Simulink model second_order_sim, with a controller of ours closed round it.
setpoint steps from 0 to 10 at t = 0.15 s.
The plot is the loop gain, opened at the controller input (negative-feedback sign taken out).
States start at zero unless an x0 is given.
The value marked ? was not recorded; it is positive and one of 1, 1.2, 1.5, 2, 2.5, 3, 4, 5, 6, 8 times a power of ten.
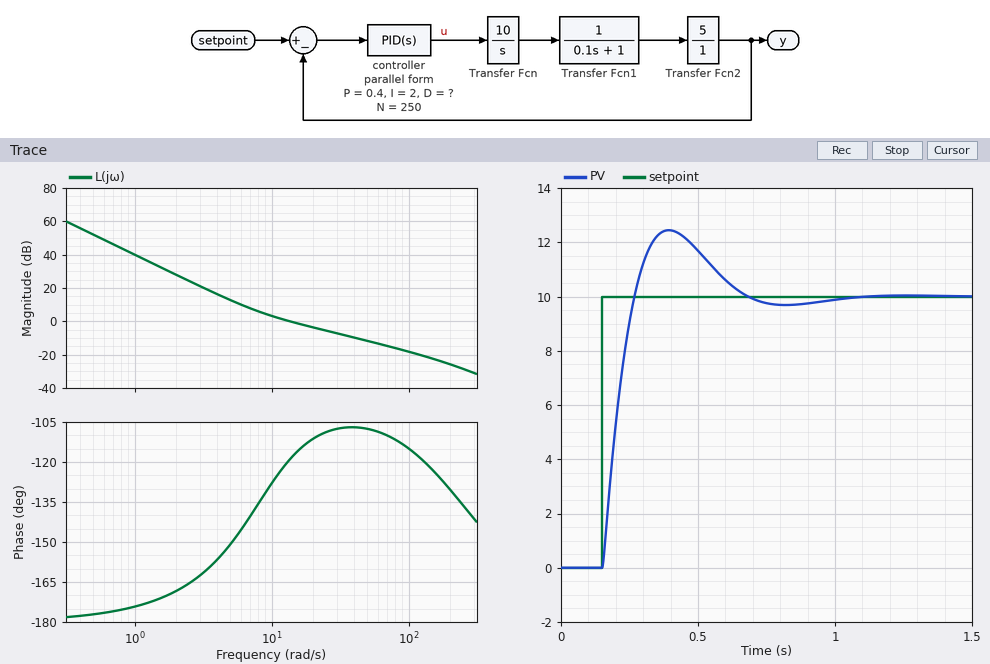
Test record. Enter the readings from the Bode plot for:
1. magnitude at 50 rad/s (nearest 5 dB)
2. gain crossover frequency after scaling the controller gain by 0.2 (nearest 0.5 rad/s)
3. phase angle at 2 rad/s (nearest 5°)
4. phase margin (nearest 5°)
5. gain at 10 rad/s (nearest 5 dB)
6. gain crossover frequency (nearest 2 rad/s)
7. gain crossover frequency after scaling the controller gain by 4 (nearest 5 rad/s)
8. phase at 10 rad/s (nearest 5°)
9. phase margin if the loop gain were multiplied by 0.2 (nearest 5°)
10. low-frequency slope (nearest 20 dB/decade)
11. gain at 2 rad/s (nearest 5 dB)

-10 dB
4.5 rad/s
-170°
60°
5 dB
14 rad/s
50 rad/s
-130°
25°
-40 dB/decade
30 dB
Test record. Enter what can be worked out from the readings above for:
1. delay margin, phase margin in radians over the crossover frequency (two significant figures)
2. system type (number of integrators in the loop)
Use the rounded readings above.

0.075 s
2
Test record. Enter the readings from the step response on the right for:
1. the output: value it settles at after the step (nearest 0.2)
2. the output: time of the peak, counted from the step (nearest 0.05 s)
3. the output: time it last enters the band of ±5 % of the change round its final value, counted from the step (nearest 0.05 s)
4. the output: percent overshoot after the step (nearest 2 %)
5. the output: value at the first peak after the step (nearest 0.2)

10.0
0.25 s
0.45 s
24 %
12.4
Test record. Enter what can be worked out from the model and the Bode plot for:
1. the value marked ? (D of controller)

0.025
